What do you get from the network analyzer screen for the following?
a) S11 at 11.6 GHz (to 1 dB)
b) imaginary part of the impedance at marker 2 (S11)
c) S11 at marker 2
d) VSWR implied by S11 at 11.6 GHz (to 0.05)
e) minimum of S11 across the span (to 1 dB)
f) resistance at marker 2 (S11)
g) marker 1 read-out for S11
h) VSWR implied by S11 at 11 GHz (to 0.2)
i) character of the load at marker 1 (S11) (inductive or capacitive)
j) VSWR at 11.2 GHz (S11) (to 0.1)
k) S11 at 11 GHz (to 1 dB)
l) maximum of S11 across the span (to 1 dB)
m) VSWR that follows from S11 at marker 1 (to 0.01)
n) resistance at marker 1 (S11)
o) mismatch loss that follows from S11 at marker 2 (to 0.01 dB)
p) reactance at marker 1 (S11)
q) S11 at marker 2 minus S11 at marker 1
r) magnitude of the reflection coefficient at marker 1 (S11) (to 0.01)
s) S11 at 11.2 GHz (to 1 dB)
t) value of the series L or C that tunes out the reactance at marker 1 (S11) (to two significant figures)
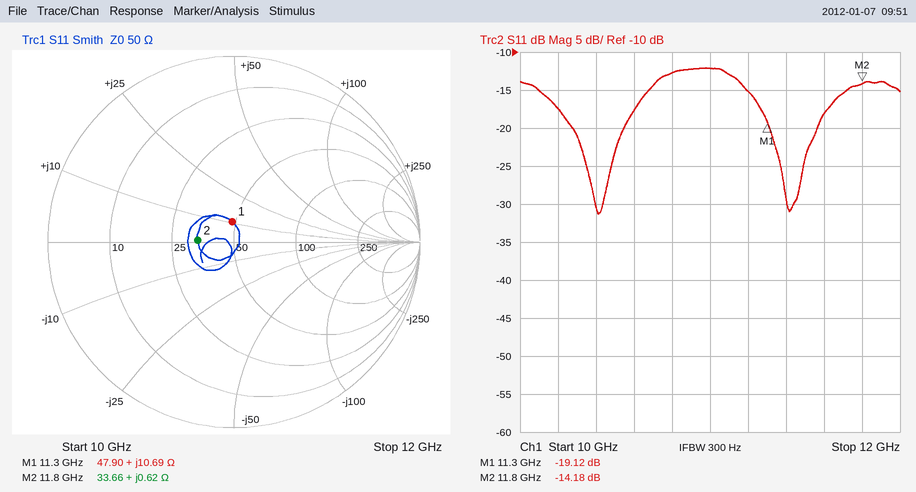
-18 dB
+0.62 Ω
-14.18 dB
1.30
-31 dB
33.66 Ω
-19.12 dB
1.6
inductive
1.4
-12 dB
-12 dB
1.25
47.90 Ω
0.17 dB
+10.69 Ω
4.94 dB
0.11
-15 dB
1.3 pF
